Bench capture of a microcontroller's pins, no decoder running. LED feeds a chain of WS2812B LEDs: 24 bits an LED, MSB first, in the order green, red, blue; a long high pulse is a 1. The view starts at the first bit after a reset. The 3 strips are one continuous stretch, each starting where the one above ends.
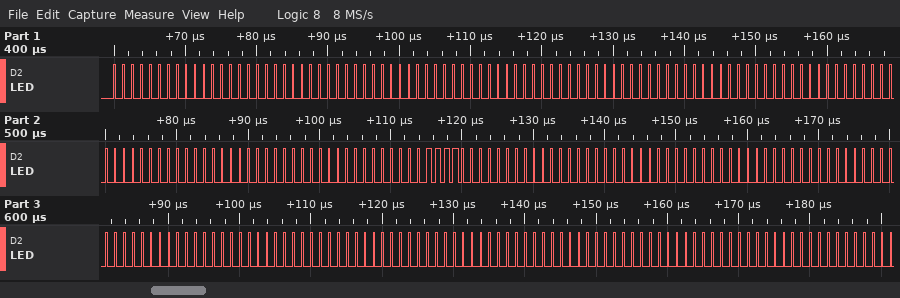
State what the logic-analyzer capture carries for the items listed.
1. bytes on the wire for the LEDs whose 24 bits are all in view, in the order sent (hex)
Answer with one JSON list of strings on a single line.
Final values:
["00 00 00 00 00 00 00 00 00 00 00 00 00 00 00 0F 00 00 00 00 00 00 00 00 00 00 00 00 00 00 00 00 00"]
